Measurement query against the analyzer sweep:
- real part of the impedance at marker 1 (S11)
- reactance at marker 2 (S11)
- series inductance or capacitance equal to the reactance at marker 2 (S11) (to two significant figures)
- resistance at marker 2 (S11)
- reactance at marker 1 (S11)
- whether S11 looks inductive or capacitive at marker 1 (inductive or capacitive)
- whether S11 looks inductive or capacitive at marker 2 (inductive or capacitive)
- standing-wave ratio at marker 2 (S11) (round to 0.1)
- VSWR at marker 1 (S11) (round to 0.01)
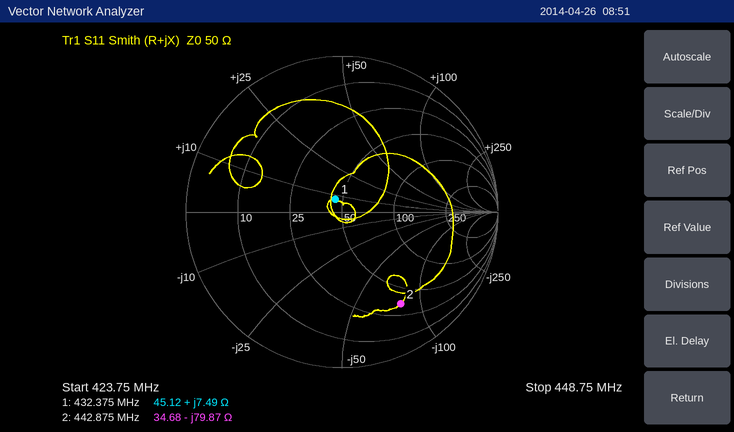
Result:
45.12 Ω
-79.87 Ω
4.5 pF
34.68 Ω
+7.49 Ω
inductive
capacitive
5.6
1.21
